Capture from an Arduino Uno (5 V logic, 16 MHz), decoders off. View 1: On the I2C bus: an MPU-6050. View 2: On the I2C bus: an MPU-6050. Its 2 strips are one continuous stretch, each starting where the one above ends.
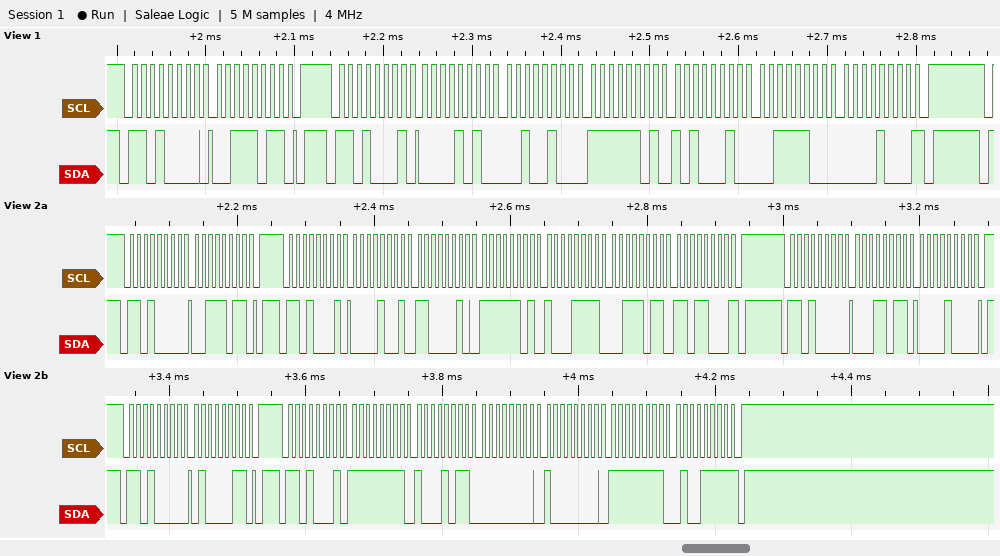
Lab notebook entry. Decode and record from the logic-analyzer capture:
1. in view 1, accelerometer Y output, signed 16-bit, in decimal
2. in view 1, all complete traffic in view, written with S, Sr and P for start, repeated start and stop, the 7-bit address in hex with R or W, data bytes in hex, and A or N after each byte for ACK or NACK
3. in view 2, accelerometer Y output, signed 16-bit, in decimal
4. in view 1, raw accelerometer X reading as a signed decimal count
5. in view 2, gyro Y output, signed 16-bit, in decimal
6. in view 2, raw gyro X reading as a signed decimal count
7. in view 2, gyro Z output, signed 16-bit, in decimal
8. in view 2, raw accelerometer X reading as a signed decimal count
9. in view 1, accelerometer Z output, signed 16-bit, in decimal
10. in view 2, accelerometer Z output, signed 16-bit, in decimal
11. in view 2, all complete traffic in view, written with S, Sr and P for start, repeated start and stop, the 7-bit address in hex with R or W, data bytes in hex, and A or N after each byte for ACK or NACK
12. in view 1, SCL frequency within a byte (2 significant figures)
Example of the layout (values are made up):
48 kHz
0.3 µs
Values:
-606
S 68W A 3B A P S 68R A 0A A 24 A FD A A2 A 3C A 08 N P
-625
2596
128
-117
-177
2498
15368
15320
S 68W A 3B A P S 68R A 09 A C2 A FD A 8F A 3B A D8 N P S 68W A 1B A 08 A P S 68W A 43 A P S 68R A FF A 8B A 00 A 80 A FF A 4F N P
100 kHz
